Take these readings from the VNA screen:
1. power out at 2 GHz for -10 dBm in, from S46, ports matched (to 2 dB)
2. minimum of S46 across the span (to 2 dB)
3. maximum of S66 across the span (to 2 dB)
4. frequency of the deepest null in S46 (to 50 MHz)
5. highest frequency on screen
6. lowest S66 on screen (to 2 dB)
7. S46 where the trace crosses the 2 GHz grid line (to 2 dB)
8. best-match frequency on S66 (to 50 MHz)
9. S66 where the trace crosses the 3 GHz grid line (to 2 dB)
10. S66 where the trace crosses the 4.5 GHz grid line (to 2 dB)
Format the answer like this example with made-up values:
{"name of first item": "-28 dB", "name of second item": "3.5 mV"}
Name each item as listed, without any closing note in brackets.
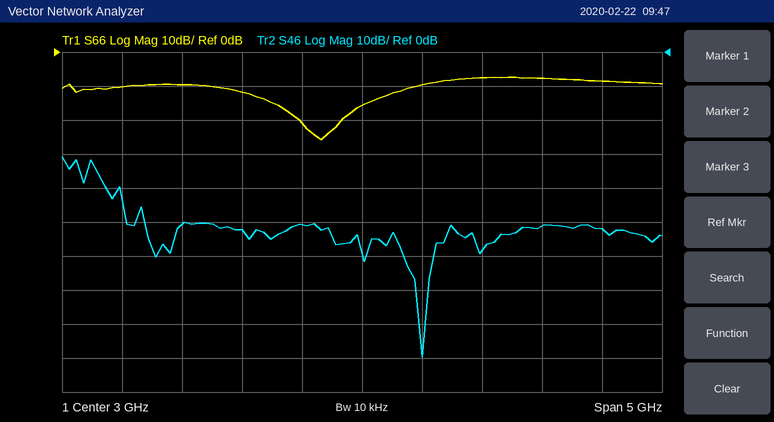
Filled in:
{"power out at 2 GHz for -10 dBm in, from S46, ports matched": "-62 dBm", "minimum of S46 across the span": "-90 dB", "maximum of S66 across the span": "-8 dB", "frequency of the deepest null in S46": "3.50 GHz", "highest frequency on screen": "5.5 GHz", "lowest S66 on screen": "-26 dB", "S46 where the trace crosses the 2 GHz grid line": "-52 dB", "best-match frequency on S66": "2.65 GHz", "S66 where the trace crosses the 3 GHz grid line": "-16 dB", "S66 where the trace crosses the 4.5 GHz grid line": "-8 dB"}
